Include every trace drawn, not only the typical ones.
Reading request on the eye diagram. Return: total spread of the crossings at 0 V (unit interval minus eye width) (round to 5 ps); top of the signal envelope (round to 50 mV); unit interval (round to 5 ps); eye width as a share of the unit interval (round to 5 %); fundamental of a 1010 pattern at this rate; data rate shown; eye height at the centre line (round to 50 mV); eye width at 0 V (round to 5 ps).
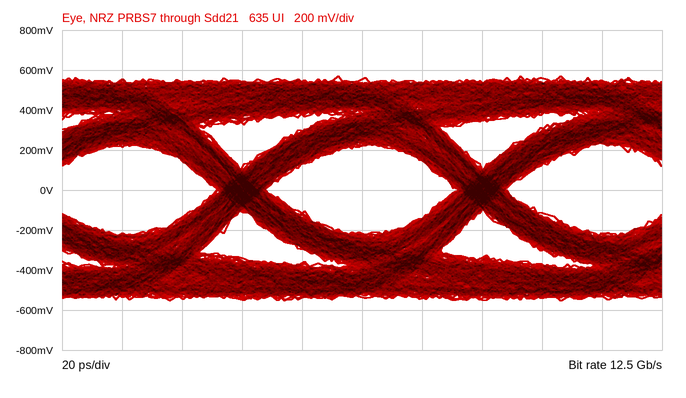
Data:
15 ps
550 mV
80 ps
80 %
6.25 GHz
12.5 Gb/s
450 mV
65 ps
